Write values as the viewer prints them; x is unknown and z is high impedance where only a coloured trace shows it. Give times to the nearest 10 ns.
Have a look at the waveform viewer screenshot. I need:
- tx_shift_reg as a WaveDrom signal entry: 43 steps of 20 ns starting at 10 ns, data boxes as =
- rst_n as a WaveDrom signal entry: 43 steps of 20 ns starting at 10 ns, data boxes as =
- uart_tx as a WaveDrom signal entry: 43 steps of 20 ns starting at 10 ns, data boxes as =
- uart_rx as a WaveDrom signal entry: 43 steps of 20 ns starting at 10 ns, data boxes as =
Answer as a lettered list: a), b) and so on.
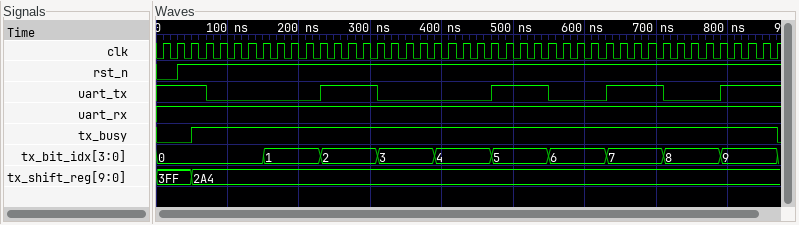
a) {name: 'tx_shift_reg', wave: '=.=........................................', data: '3FF 2A4'}
b) {name: 'rst_n', wave: '01.........................................'}
c) {name: 'uart_tx', wave: '1..0.......1...0.......1...0...1...0...1...'}
d) {name: 'uart_rx', wave: '1..........................................'}
